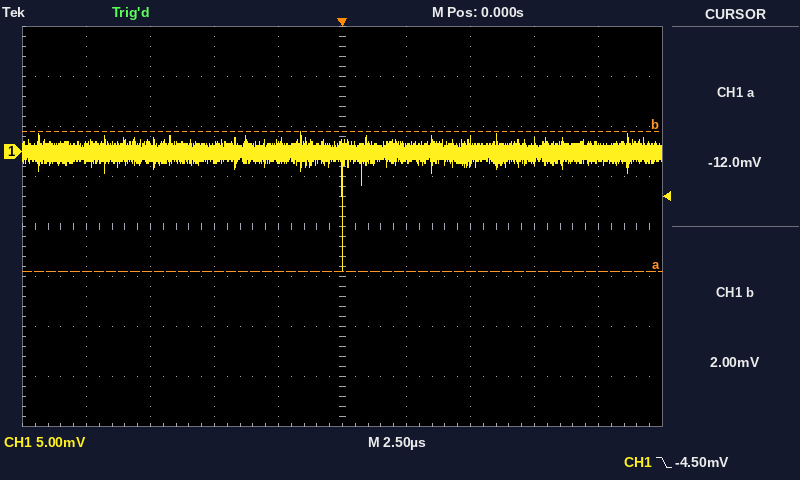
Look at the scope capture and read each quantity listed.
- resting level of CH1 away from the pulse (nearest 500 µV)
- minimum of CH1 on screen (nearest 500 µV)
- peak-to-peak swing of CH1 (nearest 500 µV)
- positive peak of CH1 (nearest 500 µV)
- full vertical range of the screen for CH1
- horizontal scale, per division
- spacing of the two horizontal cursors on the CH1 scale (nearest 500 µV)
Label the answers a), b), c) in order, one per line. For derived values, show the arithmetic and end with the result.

a) 0.0 mV
b) -12.0 mV
c) 2.0 mV − (-12.0 mV) = 14.0 mV
d) 2.0 mV
e) 40 mV
f) 2.5 µs
g) 14.0 mV
